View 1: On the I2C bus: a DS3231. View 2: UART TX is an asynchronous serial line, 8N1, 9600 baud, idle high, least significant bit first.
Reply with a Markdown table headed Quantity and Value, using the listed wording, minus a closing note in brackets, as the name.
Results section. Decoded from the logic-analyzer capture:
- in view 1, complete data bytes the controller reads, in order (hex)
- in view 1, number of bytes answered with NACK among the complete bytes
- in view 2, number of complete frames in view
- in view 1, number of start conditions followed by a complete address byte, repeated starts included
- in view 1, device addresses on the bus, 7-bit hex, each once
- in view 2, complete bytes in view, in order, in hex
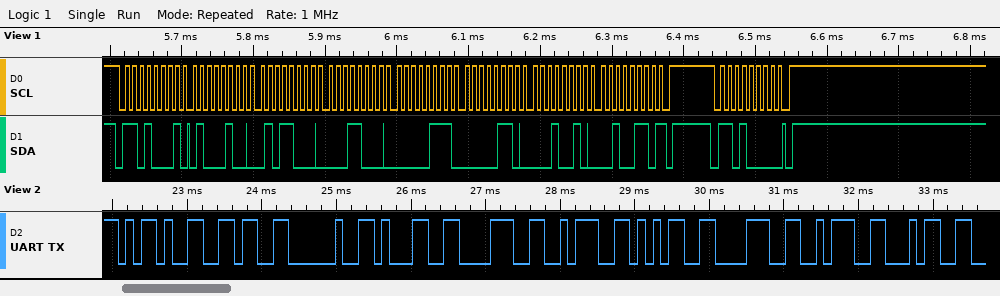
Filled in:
| Quantity | Value |
|---|---|
| in view 1, complete data bytes the controller reads, in order | 44 58 18 07 06 12 26 |
| in view 1, number of bytes answered with NACK among the complete bytes | 1 |
| in view 2, number of complete frames in view | 10 |
| in view 1, number of start conditions followed by a complete address byte, repeated starts included | 2 |
| in view 1, device addresses on the bus, 7-bit hex, each once | 0x68 |
| in view 2, complete bytes in view, in order, in hex | 0x2D 0x36 0x20 0x31 0x38 0x3A 0x35 0x38 0x3A 0x34 |
